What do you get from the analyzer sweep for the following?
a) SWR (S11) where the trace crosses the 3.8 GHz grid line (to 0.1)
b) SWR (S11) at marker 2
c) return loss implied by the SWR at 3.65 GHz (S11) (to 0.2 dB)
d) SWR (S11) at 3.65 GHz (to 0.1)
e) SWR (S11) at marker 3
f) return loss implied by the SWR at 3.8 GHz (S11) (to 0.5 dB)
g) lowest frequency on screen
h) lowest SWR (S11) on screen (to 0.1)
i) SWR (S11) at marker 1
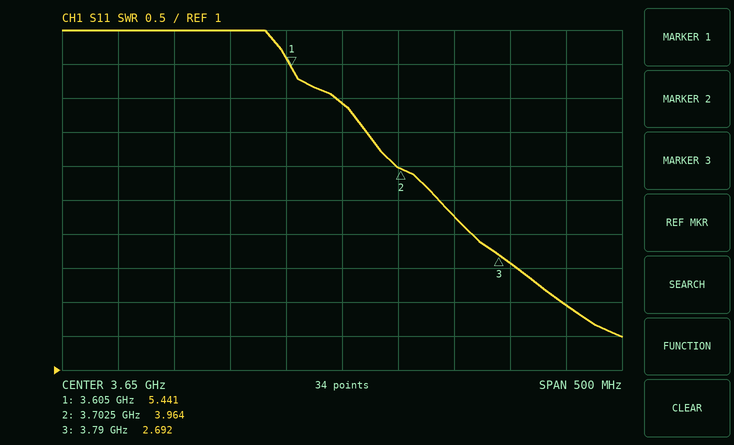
2.6
3.964
3.6 dB
4.9
2.692
7.0 dB
3.4 GHz
1.5
5.441
